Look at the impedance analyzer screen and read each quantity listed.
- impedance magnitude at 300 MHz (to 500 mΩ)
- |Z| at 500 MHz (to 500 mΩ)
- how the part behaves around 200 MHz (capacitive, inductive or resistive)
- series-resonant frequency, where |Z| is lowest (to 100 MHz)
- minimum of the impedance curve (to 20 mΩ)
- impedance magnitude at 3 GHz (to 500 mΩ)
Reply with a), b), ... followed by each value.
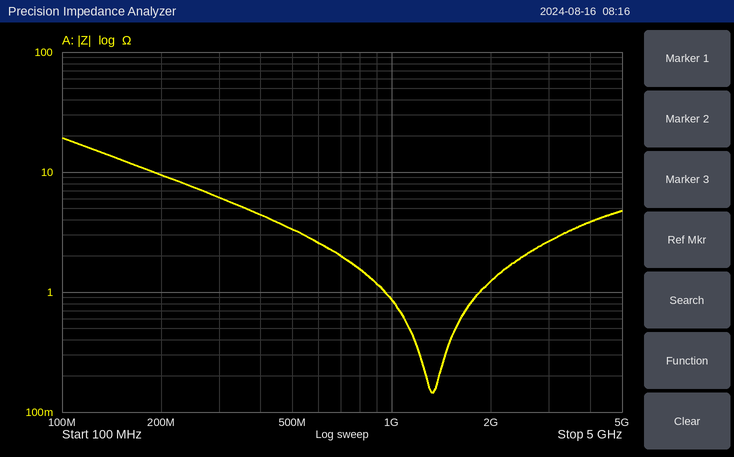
a) 6.0 Ω
b) 3.5 Ω
c) capacitive
d) 1.3 GHz
e) 140 mΩ
f) 2.5 Ω
